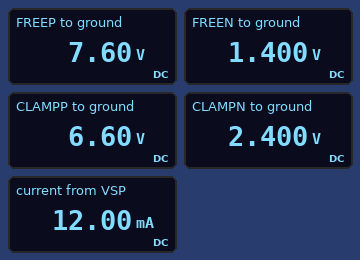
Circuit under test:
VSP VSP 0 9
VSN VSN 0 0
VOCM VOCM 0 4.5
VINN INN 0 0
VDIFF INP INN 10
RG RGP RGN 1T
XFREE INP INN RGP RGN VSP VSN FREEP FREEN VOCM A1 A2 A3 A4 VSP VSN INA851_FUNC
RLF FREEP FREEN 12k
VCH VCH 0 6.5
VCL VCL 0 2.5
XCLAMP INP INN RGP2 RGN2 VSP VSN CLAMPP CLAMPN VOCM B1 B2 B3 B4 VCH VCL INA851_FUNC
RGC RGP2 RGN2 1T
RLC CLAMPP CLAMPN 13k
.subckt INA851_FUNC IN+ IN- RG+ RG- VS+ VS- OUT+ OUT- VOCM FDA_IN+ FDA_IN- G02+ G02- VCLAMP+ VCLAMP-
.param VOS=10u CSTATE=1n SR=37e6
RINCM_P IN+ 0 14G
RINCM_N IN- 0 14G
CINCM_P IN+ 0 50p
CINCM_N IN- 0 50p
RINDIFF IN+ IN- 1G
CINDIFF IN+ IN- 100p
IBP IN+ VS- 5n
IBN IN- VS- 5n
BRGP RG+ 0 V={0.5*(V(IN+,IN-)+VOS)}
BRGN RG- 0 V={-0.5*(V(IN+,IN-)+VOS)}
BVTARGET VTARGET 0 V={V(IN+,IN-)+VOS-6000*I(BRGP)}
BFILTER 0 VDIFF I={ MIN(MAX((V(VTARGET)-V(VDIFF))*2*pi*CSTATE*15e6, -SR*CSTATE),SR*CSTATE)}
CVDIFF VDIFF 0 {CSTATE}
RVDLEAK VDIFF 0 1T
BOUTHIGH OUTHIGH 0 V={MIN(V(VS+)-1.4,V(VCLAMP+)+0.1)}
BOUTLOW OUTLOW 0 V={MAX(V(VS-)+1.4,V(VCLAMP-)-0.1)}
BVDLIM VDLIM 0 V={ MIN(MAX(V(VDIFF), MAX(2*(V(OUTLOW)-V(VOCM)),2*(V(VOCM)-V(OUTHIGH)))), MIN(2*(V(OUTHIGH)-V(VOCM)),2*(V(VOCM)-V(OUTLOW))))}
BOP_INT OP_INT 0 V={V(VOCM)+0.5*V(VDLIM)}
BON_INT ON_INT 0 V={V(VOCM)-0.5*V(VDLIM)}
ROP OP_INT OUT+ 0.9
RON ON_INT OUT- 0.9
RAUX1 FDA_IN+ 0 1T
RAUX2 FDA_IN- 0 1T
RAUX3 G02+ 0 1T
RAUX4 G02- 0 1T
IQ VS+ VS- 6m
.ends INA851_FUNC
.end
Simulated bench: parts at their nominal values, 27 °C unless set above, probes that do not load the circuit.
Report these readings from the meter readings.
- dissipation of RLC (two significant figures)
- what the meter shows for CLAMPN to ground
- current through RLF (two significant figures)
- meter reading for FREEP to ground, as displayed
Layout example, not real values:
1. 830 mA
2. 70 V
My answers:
1. 1.4 mW
2. 2.400 V
3. 520 µA
4. 7.60 V
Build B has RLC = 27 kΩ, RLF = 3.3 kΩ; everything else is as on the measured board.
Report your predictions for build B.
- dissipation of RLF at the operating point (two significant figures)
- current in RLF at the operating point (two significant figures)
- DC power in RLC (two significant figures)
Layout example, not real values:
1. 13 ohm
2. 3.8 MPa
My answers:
1. 12 mW
2. 1.9 mA
3. 650 µW
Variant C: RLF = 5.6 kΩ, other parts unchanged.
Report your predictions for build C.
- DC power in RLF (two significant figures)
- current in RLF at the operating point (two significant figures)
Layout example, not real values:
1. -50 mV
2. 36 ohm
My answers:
1. 6.9 mW
2. 1.1 mA
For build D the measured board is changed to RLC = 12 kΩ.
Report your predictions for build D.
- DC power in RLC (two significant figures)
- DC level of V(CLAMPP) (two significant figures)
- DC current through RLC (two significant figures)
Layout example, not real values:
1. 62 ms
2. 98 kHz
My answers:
1. 1.5 mW
2. 6.6 V
3. 350 µA
